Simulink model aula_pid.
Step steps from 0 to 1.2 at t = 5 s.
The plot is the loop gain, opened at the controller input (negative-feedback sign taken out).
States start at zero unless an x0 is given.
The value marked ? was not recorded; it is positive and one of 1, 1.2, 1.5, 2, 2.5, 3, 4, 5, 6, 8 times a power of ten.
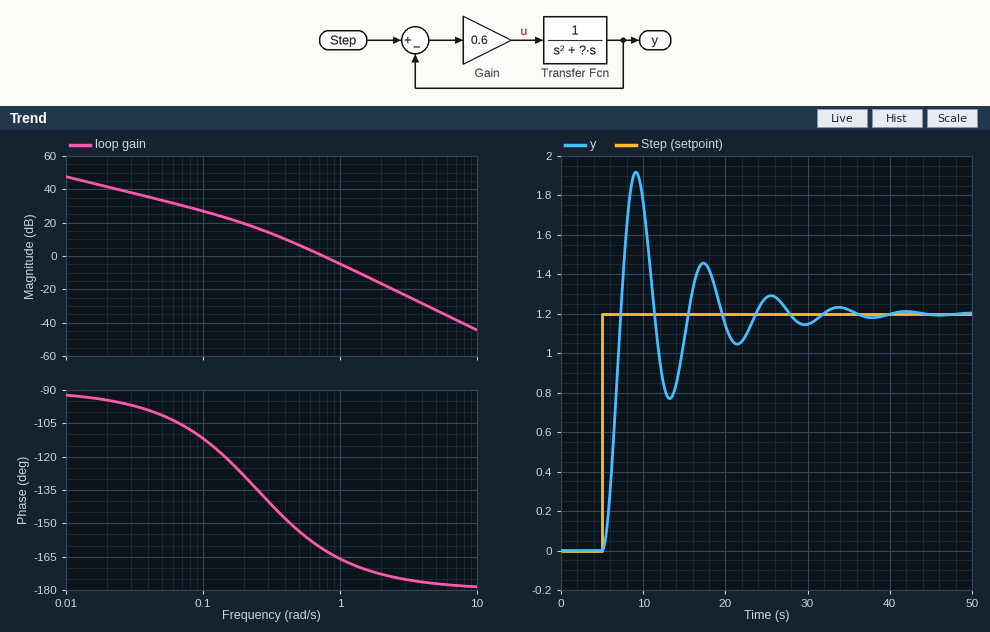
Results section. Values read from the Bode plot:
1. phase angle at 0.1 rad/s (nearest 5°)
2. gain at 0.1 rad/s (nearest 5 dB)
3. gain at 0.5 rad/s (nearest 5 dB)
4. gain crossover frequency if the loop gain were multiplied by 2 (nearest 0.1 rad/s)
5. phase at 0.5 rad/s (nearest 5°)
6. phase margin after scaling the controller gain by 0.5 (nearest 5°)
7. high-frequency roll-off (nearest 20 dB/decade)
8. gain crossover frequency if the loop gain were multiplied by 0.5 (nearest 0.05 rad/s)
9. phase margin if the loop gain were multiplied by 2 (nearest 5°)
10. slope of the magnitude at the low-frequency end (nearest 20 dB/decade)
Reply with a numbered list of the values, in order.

1. -110°
2. 25 dB
3. 5 dB
4. 1.1 rad/s
5. -155°
6. 25°
7. -40 dB/decade
8. 0.50 rad/s
9. 15°
10. -20 dB/decade
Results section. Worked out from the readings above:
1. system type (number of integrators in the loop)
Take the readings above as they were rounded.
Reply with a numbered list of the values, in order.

1. 1
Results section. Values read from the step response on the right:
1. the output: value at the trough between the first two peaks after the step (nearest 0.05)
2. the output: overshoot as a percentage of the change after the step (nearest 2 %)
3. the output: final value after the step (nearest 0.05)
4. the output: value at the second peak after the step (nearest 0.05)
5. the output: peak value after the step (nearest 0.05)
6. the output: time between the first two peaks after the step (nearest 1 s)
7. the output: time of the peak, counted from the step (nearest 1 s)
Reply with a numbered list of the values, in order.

1. 0.75
2. 60 %
3. 1.20
4. 1.45
5. 1.90
6. 8 s
7. 4 s
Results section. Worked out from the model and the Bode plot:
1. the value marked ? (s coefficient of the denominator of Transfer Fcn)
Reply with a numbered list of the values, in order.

1. 0.25
